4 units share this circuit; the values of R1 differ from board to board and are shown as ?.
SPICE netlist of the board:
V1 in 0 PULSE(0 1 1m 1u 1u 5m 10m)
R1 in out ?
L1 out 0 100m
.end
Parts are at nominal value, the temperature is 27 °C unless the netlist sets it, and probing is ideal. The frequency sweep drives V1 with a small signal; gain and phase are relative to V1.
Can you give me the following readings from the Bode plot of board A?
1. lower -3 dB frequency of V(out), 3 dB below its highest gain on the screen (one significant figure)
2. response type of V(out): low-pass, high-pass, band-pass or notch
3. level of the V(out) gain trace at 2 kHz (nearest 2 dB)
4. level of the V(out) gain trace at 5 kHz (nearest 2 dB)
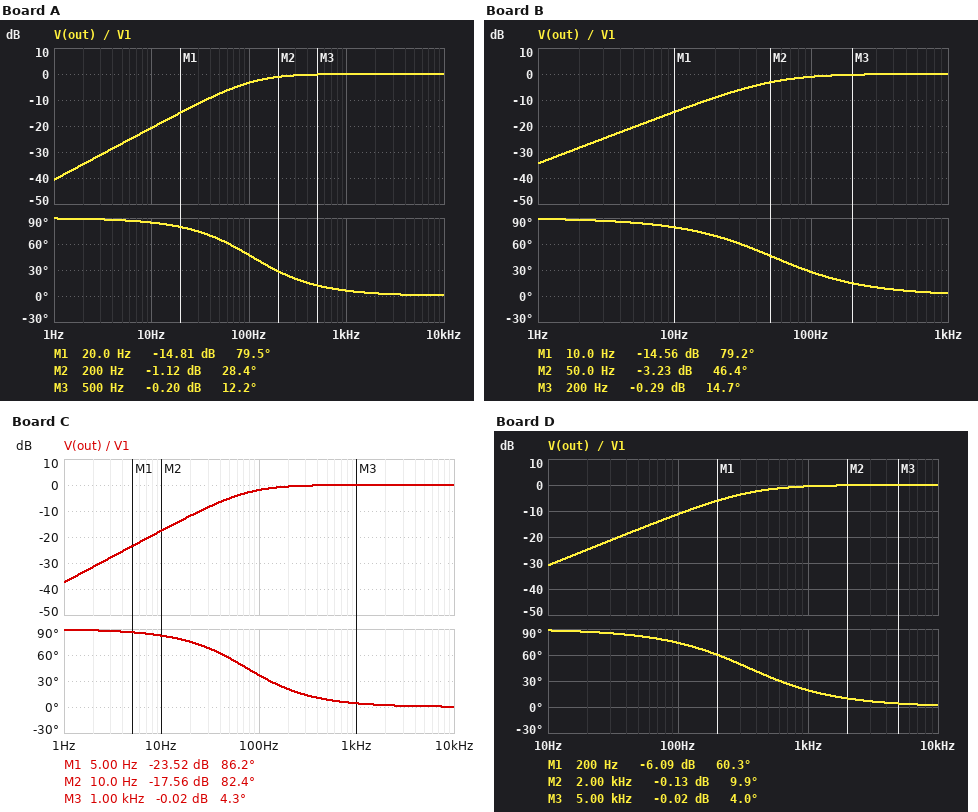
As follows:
100 Hz
high-pass
0 dB
0 dB
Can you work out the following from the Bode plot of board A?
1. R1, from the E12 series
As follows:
68 Ω
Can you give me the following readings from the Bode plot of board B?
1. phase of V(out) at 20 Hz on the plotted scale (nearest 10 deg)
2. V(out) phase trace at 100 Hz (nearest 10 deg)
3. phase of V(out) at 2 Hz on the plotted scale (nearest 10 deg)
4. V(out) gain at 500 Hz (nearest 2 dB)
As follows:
70 deg
30 deg
90 deg
0 dB
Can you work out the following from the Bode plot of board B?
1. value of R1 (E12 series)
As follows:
33 Ω
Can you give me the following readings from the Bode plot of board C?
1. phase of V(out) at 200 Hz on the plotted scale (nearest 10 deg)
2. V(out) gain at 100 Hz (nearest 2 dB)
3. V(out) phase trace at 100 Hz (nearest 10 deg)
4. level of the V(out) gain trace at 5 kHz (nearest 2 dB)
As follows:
20 deg
-2 dB
40 deg
0 dB
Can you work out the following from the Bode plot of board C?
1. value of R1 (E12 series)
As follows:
47 Ω
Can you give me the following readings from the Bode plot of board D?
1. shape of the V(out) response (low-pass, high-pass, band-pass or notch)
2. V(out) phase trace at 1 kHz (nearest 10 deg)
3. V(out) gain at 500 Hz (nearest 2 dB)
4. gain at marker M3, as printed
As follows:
high-pass
20 deg
-2 dB
-0.02 dB
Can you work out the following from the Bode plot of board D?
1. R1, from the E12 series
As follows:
220 Ω
